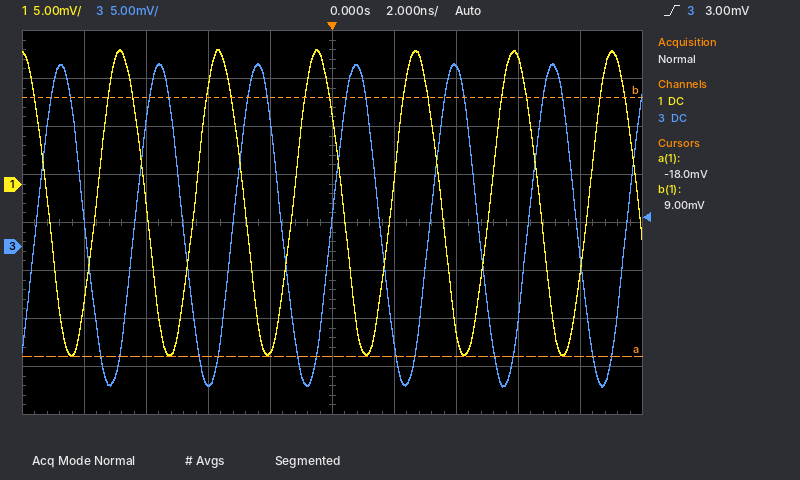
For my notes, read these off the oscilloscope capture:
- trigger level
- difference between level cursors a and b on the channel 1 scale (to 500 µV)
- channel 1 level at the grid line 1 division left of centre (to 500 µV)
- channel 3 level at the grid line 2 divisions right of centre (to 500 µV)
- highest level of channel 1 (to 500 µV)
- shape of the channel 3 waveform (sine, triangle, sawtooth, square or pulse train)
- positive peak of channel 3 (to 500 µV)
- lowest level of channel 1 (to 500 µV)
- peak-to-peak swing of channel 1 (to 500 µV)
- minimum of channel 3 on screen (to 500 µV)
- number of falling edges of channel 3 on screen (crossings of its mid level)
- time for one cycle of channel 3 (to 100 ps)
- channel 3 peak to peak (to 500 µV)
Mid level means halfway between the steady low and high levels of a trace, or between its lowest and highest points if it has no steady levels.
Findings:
3.00 mV
27.0 mV
-17.5 mV
18.5 mV
14.0 mV
sine
19.0 mV
-18.0 mV
32.0 mV
-14.5 mV
6
3.2 ns
33.5 mV
